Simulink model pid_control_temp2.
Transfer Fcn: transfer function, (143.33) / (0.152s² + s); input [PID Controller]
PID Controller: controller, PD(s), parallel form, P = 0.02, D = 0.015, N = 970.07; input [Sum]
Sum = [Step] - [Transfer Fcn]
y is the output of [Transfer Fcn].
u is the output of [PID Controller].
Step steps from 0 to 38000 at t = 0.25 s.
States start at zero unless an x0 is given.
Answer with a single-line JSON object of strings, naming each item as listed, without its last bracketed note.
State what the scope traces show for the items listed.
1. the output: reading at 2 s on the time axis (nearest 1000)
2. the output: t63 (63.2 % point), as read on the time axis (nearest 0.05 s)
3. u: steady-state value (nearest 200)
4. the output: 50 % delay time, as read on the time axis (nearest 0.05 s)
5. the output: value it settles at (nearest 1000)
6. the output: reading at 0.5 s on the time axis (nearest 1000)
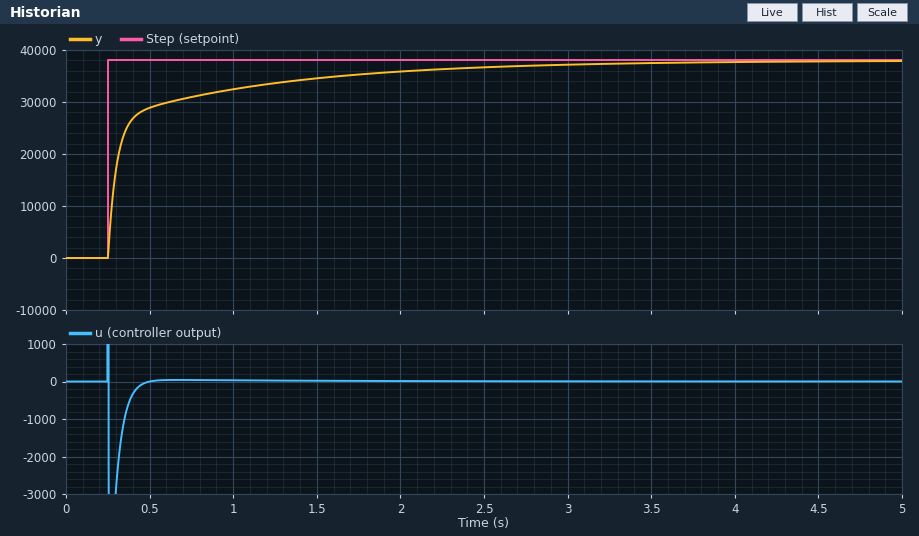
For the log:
{"the output: reading at 2 s on the time axis": "36000", "the output: t63 (63.2 % point), as read on the time axis": "0.35 s", "u: steady-state value": "0", "the output: 50 % delay time, as read on the time axis": "0.30 s", "the output: value it settles at": "38000", "the output: reading at 0.5 s on the time axis": "29000"}
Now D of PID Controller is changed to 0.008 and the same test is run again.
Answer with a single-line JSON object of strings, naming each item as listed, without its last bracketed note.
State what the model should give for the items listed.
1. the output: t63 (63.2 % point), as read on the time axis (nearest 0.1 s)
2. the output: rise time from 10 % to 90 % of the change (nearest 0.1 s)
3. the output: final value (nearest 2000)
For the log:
{"the output: t63 (63.2 % point), as read on the time axis": "0.5 s", "the output: rise time from 10 % to 90 % of the change": "1.0 s", "the output: final value": "38000"}
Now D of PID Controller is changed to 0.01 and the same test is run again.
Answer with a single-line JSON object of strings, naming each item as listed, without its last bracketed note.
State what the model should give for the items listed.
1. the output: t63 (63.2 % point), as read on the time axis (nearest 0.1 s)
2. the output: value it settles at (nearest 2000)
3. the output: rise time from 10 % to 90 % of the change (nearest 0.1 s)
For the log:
{"the output: t63 (63.2 % point), as read on the time axis": "0.4 s", "the output: value it settles at": "38000", "the output: rise time from 10 % to 90 % of the change": "1.1 s"}
